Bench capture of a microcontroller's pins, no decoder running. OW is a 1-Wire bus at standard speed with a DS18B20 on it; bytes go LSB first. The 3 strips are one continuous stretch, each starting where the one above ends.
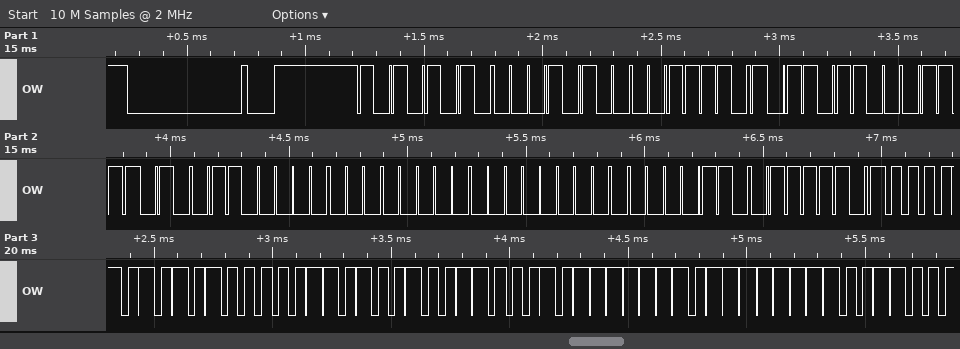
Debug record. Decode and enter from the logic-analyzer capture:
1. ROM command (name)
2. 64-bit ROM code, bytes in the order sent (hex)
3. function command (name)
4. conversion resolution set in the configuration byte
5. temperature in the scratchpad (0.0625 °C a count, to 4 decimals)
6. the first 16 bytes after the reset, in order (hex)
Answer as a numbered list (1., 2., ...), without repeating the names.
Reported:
1. Match ROM
2. 28 BC 36 5E 06 00 00 60
3. Read Scratchpad
4. 12 bits
5. 85.0000 °C
6. 55 28 BC 36 5E 06 00 00 60 BE 50 05 4B 46 7F FF
